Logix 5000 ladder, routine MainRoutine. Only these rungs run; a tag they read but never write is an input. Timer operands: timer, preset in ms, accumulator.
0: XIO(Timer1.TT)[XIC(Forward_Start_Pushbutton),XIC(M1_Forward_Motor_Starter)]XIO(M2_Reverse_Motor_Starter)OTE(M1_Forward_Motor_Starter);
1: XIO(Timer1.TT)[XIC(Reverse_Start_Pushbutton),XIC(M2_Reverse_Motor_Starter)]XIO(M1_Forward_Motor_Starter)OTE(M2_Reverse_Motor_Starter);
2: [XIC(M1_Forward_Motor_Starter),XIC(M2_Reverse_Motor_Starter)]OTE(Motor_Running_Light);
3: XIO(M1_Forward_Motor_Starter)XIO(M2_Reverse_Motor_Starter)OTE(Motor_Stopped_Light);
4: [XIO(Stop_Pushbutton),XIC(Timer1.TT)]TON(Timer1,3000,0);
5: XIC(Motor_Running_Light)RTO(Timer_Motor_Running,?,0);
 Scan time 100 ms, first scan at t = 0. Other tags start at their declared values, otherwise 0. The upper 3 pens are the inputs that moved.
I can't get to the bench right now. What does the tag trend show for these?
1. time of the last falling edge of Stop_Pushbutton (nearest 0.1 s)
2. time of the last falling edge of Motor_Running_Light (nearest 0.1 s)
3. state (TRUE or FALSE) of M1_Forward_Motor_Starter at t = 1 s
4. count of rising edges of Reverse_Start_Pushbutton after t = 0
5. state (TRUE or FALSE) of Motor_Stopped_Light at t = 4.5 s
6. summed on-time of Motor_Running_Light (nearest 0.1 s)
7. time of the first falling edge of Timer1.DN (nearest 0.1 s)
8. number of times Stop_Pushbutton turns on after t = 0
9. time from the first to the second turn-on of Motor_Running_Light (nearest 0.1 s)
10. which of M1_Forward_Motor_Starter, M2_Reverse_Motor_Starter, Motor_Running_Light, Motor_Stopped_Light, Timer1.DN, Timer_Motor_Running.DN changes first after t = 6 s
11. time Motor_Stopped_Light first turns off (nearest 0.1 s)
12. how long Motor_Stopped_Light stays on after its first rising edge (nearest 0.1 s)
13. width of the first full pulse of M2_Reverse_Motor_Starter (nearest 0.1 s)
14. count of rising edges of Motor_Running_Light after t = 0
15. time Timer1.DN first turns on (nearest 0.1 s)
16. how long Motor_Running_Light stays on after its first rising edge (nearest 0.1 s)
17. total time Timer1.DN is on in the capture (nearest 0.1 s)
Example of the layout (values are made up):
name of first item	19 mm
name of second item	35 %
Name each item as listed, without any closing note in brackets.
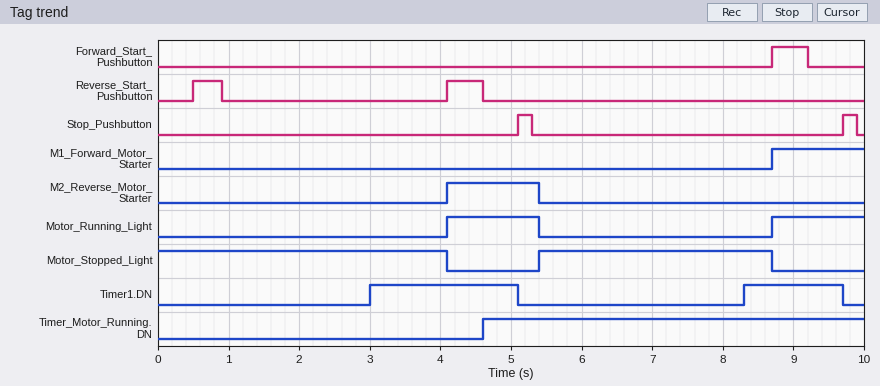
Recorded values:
time of the last falling edge of Stop_Pushbutton	9.9 s
time of the last falling edge of Motor_Running_Light	5.4 s
state (TRUE or FALSE) of M1_Forward_Motor_Starter at t = 1 s	FALSE
count of rising edges of Reverse_Start_Pushbutton after t = 0	2
state (TRUE or FALSE) of Motor_Stopped_Light at t = 4.5 s	FALSE
summed on-time of Motor_Running_Light	2.6 s
time of the first falling edge of Timer1.DN	5.1 s
number of times Stop_Pushbutton turns on after t = 0	2
time from the first to the second turn-on of Motor_Running_Light	4.6 s
which of M1_Forward_Motor_Starter, M2_Reverse_Motor_Starter, Motor_Running_Light, Motor_Stopped_Light, Timer1.DN, Timer_Motor_Running.DN changes first after t = 6 s	Timer1.DN
time Motor_Stopped_Light first turns off	4.1 s
how long Motor_Stopped_Light stays on after its first rising edge	3.3 s
width of the first full pulse of M2_Reverse_Motor_Starter	1.3 s
count of rising edges of Motor_Running_Light after t = 0	2
time Timer1.DN first turns on	3.0 s
how long Motor_Running_Light stays on after its first rising edge	1.3 s
total time Timer1.DN is on in the capture	3.5 s
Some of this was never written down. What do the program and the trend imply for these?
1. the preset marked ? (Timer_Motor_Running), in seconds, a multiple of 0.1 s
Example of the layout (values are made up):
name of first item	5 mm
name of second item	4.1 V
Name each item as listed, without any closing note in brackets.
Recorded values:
the preset marked ? (Timer_Motor_Running), in seconds, a multiple of 0.1 s	0.5 s
